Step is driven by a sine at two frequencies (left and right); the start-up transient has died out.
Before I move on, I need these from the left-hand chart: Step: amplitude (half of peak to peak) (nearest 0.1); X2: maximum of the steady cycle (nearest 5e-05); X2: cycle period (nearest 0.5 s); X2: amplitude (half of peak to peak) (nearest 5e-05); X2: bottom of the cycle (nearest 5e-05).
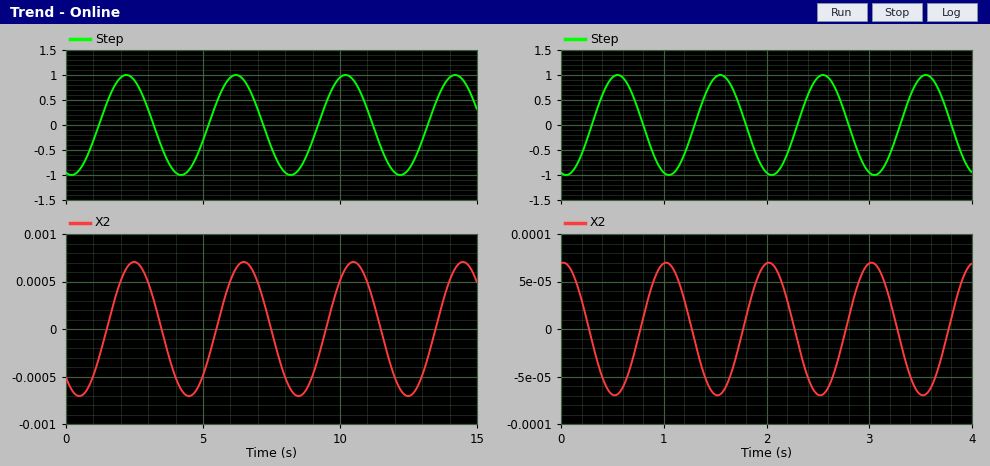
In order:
1.0
0.00070
4.0 s
0.00070
-0.00070
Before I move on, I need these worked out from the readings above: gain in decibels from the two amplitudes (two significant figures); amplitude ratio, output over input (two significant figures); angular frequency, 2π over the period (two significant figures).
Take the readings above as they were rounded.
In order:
-63 dB
0.00070
1.6 rad/s
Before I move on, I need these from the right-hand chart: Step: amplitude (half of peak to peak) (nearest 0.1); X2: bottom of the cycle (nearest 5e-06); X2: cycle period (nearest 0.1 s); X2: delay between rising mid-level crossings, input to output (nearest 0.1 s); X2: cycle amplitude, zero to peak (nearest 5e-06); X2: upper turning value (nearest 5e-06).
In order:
1.0
-0.000070
1.0 s
0.5 s
0.000070
0.000070
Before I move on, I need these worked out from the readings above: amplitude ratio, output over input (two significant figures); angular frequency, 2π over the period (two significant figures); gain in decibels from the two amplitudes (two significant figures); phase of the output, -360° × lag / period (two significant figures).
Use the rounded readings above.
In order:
0.000070
6.3 rad/s
-83 dB
-180°
